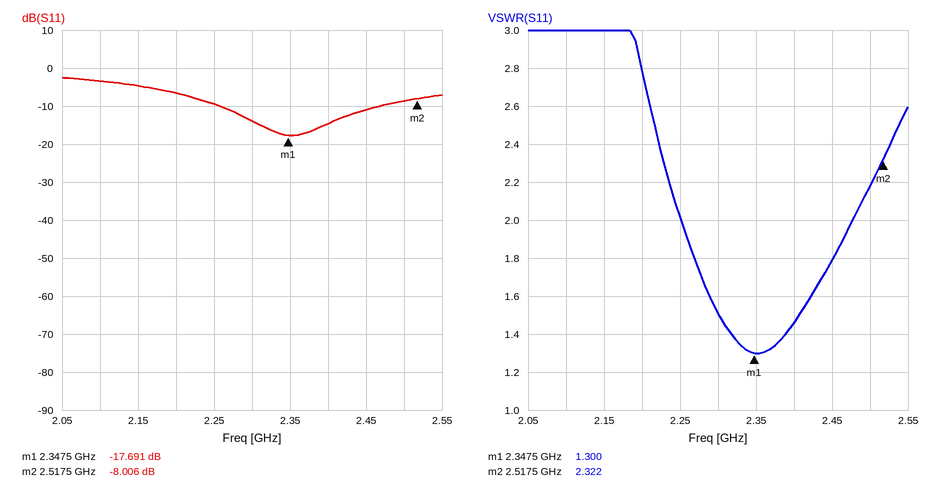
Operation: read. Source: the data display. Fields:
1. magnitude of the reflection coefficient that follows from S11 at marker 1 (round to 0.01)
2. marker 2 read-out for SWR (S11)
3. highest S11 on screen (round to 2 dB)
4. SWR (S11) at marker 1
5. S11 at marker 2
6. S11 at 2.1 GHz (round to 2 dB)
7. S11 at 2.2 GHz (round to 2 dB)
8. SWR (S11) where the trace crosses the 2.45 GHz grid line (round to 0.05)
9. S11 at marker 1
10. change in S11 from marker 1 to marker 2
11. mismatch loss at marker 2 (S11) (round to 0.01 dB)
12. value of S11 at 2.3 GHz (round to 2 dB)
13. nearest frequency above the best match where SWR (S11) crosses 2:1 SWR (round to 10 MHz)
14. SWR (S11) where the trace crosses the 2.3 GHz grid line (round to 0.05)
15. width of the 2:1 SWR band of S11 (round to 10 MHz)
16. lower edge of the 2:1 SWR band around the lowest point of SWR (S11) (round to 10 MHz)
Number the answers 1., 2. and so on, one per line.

1. 0.13
2. 2.322
3. -2 dB
4. 1.300
5. -8.006 dB
6. -4 dB
7. -6 dB
8. 1.80
9. -17.691 dB
10. 9.685 dB
11. 0.75 dB
12. -14 dB
13. 2.48 GHz
14. 1.50
15. 230 MHz
16. 2.25 GHz
